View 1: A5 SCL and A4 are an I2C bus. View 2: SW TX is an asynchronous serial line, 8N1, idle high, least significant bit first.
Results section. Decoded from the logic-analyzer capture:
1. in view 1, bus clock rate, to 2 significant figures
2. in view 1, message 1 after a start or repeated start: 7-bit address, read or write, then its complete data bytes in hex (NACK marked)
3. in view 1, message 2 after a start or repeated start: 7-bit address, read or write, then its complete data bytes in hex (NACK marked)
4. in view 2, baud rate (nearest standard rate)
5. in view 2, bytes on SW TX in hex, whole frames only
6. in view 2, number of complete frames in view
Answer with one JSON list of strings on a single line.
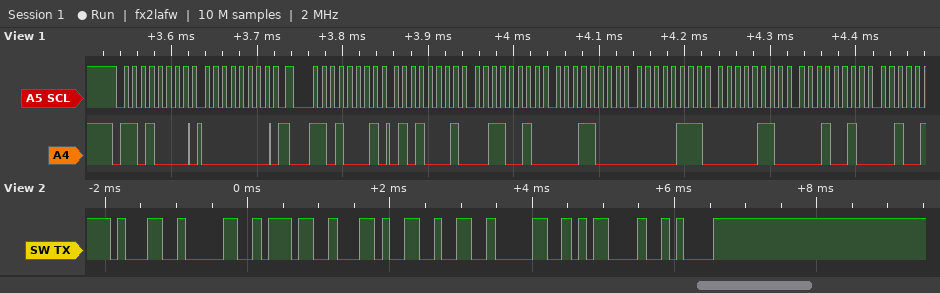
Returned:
["100 kHz", "0x68 write: 00", "0x68 read: 51 32 18 07 06 12", "9600 baud", "31 30 37 2C 32 30 0D 0A", "8"]
